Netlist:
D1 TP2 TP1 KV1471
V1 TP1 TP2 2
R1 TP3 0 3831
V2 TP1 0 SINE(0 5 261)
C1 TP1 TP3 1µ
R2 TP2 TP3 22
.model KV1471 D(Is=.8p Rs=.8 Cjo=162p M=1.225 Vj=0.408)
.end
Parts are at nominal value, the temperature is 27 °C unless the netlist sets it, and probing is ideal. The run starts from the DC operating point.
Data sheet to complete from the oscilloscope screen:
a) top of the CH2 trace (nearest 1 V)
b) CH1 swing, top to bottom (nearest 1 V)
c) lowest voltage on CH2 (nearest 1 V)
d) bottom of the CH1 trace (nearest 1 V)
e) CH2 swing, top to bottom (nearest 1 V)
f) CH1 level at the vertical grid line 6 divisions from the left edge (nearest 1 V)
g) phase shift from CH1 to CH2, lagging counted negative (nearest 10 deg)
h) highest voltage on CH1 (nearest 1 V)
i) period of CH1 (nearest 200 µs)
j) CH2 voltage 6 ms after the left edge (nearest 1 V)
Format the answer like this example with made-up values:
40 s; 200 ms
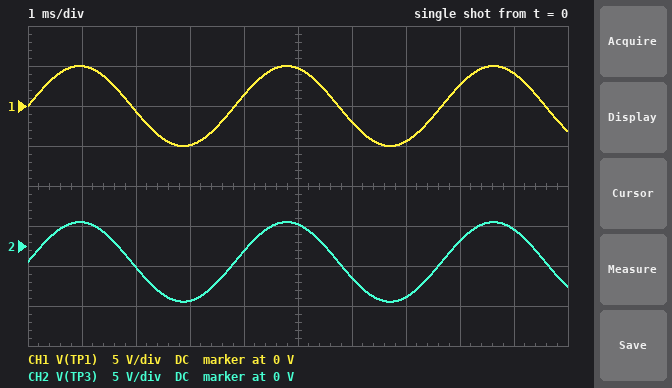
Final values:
3 V; 10 V; -7 V; -5 V; 10 V; -2 V; 0 deg; 5 V; 3.8 ms; -4 V
